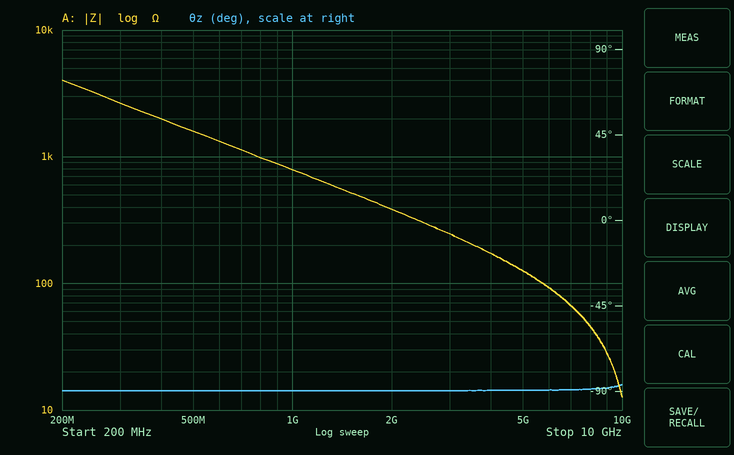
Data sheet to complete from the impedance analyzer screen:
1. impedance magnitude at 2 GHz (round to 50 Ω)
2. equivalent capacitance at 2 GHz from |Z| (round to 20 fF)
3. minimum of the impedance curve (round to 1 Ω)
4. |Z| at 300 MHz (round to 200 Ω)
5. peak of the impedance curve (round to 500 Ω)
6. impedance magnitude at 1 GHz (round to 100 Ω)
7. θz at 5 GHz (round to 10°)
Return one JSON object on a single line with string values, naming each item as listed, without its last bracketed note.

{"impedance magnitude at 2 GHz": "400 Ω", "equivalent capacitance at 2 GHz from |Z|": "200 fF", "minimum of the impedance curve": "13 Ω", "|Z| at 300 MHz": "2.6 kΩ", "peak of the impedance curve": "4.0 kΩ", "impedance magnitude at 1 GHz": "800 Ω", "θz at 5 GHz": "-90°"}
